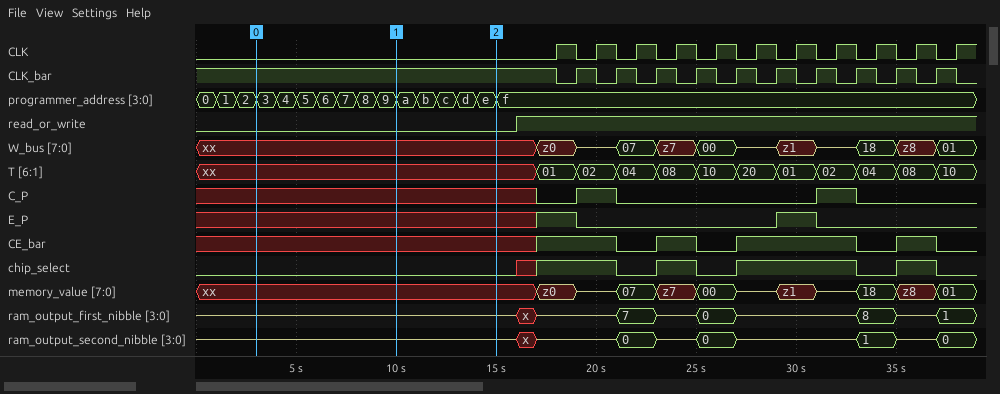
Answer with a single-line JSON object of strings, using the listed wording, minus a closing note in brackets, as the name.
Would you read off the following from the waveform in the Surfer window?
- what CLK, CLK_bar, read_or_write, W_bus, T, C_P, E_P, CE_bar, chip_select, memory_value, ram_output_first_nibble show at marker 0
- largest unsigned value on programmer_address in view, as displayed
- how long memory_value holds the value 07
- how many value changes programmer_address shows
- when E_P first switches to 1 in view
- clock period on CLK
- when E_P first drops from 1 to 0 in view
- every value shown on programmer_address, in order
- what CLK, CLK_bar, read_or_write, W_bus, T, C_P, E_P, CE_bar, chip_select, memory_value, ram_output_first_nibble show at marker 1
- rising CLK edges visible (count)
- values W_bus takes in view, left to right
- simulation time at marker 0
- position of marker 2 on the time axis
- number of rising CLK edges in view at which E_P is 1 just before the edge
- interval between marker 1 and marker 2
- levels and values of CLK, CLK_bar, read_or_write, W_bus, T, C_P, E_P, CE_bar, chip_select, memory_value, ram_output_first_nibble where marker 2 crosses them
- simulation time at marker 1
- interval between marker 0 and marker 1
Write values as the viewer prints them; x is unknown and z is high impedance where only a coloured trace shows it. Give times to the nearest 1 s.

{"what CLK, CLK_bar, read_or_write, W_bus, T, C_P, E_P, CE_bar, chip_select, memory_value, ram_output_first_nibble show at marker 0": "CLK=0, CLK_bar=1, read_or_write=0, W_bus=xx, T=xx, C_P=x, E_P=x, CE_bar=x, chip_select=0, memory_value=xx, ram_output_first_nibble=z", "largest unsigned value on programmer_address in view, as displayed": "f", "how long memory_value holds the value 07": "2 s", "how many value changes programmer_address shows": "15", "when E_P first switches to 1 in view": "17 s", "clock period on CLK": "2 s", "when E_P first drops from 1 to 0 in view": "19 s", "every value shown on programmer_address, in order": "0, 1, 2, 3, 4, 5, 6, 7, 8, 9, a, b, c, d, e, f", "what CLK, CLK_bar, read_or_write, W_bus, T, C_P, E_P, CE_bar, chip_select, memory_value, ram_output_first_nibble show at marker 1": "CLK=0, CLK_bar=1, read_or_write=0, W_bus=xx, T=xx, C_P=x, E_P=x, CE_bar=x, chip_select=0, memory_value=xx, ram_output_first_nibble=z", "rising CLK edges visible": "11", "values W_bus takes in view, left to right": "xx, z0, z, 07, z7, 00, z, z1, z, 18, z8, 01", "simulation time at marker 0": "3 s", "position of marker 2 on the time axis": "15 s", "number of rising CLK edges in view at which E_P is 1 just before the edge": "2", "interval between marker 1 and marker 2": "5 s", "levels and values of CLK, CLK_bar, read_or_write, W_bus, T, C_P, E_P, CE_bar, chip_select, memory_value, ram_output_first_nibble where marker 2 crosses them": "CLK=0, CLK_bar=1, read_or_write=0, W_bus=xx, T=xx, C_P=x, E_P=x, CE_bar=x, chip_select=0, memory_value=xx, ram_output_first_nibble=z", "simulation time at marker 1": "10 s", "interval between marker 0 and marker 1": "7 s"}
